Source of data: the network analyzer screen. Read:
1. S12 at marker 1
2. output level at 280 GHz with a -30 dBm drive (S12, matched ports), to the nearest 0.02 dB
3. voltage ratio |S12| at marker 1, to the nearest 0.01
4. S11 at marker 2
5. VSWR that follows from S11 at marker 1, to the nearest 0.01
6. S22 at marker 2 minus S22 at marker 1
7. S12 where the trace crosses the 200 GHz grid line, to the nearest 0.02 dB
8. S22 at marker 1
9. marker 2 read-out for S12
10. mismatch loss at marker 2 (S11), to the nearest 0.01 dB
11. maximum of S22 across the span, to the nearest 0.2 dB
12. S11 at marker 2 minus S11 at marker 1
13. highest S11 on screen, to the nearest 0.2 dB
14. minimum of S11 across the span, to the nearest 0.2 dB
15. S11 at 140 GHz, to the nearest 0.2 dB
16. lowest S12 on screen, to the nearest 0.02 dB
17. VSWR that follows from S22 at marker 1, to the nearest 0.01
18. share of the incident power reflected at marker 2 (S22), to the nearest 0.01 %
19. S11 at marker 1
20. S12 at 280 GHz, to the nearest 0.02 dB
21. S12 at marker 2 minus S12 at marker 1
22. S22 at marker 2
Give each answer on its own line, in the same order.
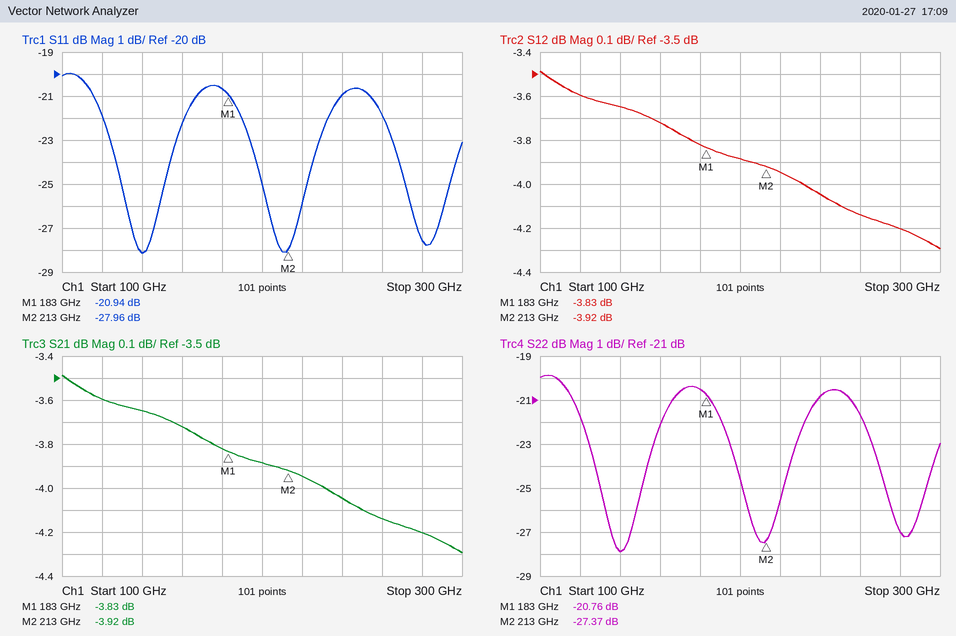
-3.83 dB
-34.20 dBm
0.64
-27.96 dB
1.20
-6.61 dB
-3.88 dB
-20.76 dB
-3.92 dB
0.01 dB
-19.8 dB
-7.02 dB
-20.0 dB
-28.2 dB
-28.2 dB
-4.30 dB
1.20
0.18 %
-20.94 dB
-4.20 dB
-0.09 dB
-27.37 dB
